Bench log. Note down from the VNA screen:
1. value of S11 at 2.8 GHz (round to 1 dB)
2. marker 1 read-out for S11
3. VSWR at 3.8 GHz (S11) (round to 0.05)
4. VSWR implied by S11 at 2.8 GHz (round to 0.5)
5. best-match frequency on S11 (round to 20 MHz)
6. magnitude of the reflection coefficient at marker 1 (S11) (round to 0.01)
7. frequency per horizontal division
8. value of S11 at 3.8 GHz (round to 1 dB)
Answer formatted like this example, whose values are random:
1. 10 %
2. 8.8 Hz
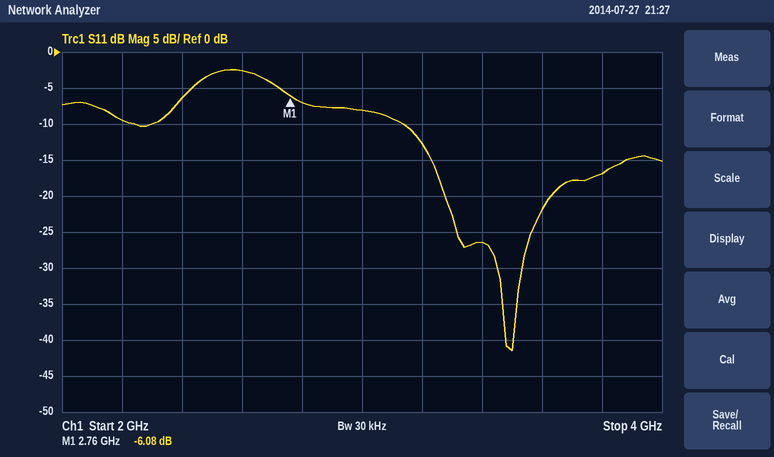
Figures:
1. -7 dB
2. -6.08 dB
3. 1.35
4. 2.5
5. 3.50 GHz
6. 0.50
7. 200 MHz
8. -17 dB
